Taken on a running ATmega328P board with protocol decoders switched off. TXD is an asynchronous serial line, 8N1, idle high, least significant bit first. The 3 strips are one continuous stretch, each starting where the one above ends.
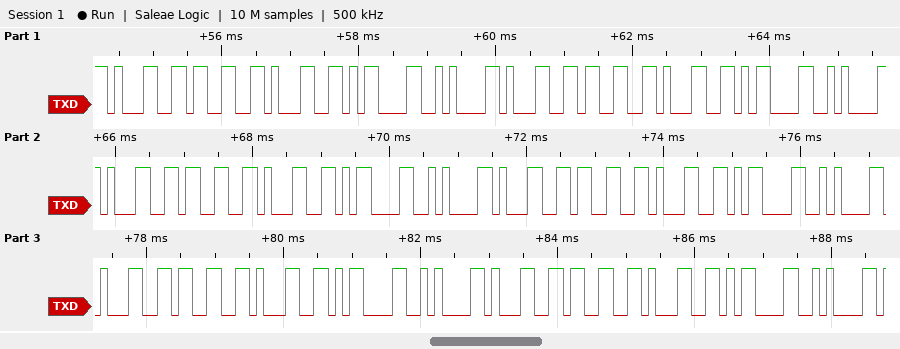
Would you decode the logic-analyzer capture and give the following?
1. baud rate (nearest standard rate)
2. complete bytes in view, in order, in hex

9600 baud
31 33 31 0D 0A 31 33 31 0D 0A 31 33 31 0D 0A 31 33 31 0D 0A 31 33 31 0D 0A 31 33 31 0D 0A
